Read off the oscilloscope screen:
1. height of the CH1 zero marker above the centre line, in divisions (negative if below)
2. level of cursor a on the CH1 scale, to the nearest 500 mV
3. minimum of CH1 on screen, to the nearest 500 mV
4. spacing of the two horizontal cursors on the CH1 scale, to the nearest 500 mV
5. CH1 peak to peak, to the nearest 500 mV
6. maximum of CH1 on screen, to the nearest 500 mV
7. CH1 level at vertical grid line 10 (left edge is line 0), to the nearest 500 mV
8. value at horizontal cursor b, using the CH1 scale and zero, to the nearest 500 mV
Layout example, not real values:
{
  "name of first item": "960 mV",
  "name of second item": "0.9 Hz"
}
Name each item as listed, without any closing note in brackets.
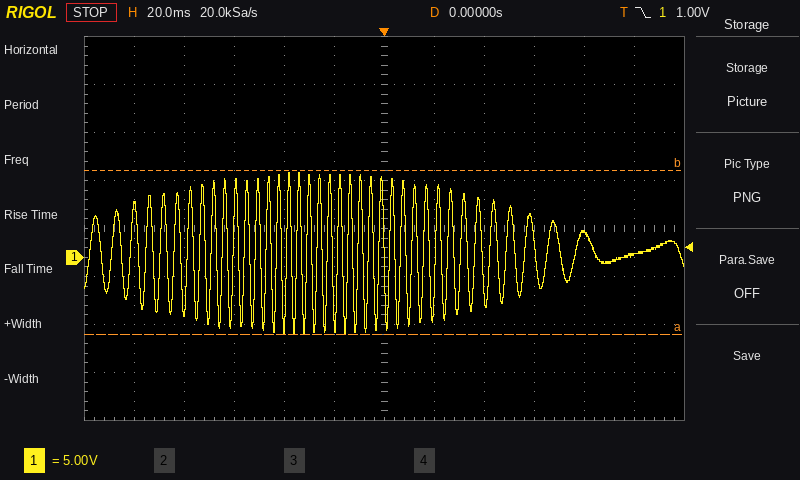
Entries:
{
  "height of the CH1 zero marker above the centre line, in divisions": "-0.6 div",
  "level of cursor a on the CH1 scale, to the nearest 500 mV": "-8.0 V",
  "minimum of CH1 on screen, to the nearest 500 mV": "-8.0 V",
  "spacing of the two horizontal cursors on the CH1 scale, to the nearest 500 mV": "17.0 V",
  "CH1 peak to peak, to the nearest 500 mV": "17.0 V",
  "maximum of CH1 on screen, to the nearest 500 mV": "9.0 V",
  "CH1 level at vertical grid line 10 (left edge is line 0), to the nearest 500 mV": "2.5 V",
  "value at horizontal cursor b, using the CH1 scale and zero, to the nearest 500 mV": "9.0 V"
}
